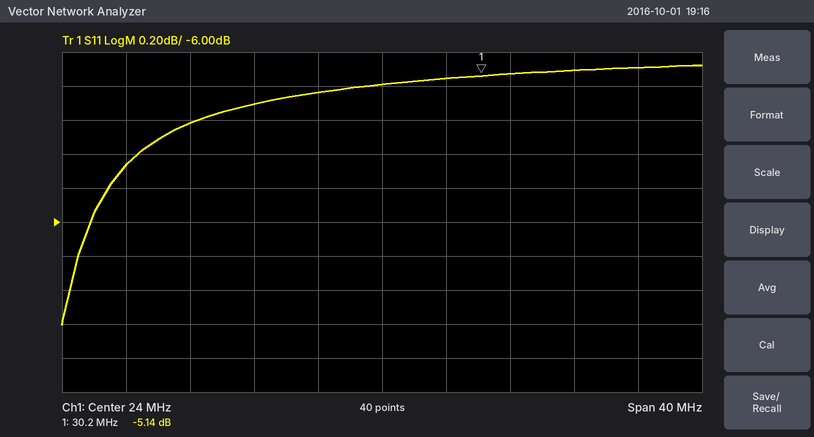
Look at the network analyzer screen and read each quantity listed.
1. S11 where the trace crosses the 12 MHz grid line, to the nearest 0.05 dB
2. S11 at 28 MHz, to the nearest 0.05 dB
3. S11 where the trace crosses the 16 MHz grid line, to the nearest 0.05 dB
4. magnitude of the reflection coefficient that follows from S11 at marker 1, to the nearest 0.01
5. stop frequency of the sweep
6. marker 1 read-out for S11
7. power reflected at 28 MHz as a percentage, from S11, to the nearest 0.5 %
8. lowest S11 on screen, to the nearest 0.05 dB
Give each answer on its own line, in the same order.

-5.40 dB
-5.15 dB
-5.30 dB
0.55
44 MHz
-5.14 dB
30.5 %
-6.60 dB
